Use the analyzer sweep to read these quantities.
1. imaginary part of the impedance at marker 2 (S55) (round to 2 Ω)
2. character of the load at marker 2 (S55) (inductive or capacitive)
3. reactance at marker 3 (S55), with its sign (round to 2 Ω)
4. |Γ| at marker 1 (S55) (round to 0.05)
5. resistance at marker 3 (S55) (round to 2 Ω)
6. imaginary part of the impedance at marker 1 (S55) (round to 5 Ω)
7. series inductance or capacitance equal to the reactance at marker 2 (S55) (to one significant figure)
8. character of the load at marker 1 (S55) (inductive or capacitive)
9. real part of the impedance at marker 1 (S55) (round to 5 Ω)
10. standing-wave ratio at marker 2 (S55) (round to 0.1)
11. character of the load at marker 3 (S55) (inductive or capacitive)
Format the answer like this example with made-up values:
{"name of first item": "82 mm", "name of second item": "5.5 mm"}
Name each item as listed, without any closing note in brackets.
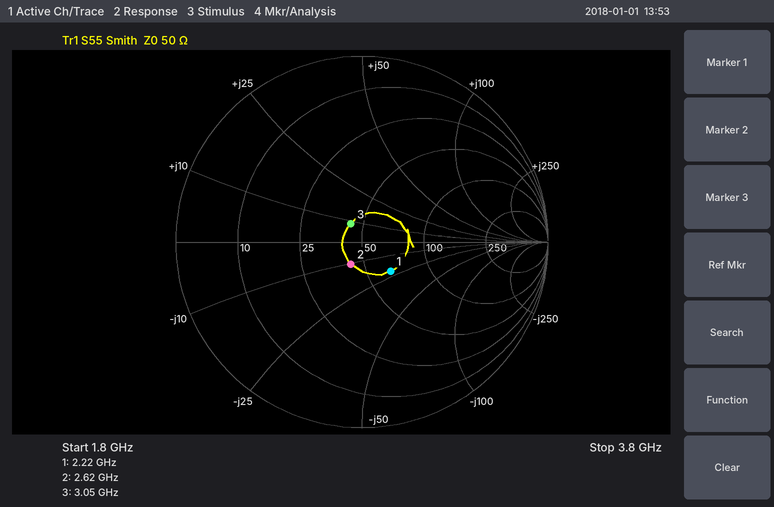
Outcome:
{"imaginary part of the impedance at marker 2 (S55)": "-10 Ω", "character of the load at marker 2 (S55)": "capacitive", "reactance at marker 3 (S55), with its sign": "+8 Ω", "|Γ| at marker 1 (S55)": "0.20", "resistance at marker 3 (S55)": "44 Ω", "imaginary part of the impedance at marker 1 (S55)": "-20 Ω", "series inductance or capacitance equal to the reactance at marker 2 (S55)": "6 pF", "character of the load at marker 1 (S55)": "capacitive", "real part of the impedance at marker 1 (S55)": "65 Ω", "standing-wave ratio at marker 2 (S55)": "1.3", "character of the load at marker 3 (S55)": "inductive"}
